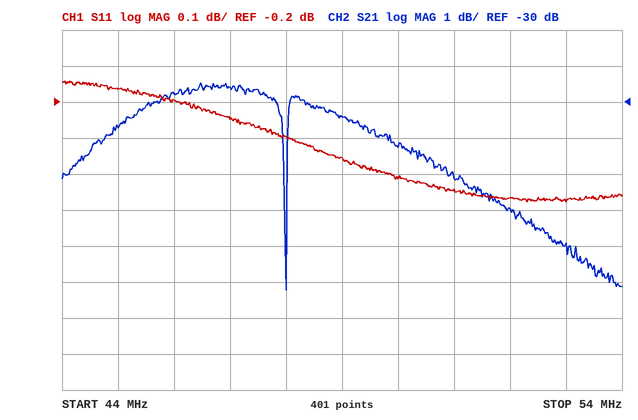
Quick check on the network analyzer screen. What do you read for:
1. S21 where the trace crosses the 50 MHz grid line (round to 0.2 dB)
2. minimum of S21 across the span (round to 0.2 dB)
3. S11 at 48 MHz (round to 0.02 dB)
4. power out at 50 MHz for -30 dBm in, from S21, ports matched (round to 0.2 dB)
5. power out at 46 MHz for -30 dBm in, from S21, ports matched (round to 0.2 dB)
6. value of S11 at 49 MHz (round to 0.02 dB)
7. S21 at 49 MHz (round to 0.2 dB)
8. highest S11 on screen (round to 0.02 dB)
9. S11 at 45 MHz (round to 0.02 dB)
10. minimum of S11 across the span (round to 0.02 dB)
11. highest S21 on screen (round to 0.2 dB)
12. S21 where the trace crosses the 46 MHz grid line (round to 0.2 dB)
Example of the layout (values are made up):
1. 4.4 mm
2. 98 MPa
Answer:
1. -31.2 dB
2. -35.2 dB
3. -0.30 dB
4. -61.2 dBm
5. -59.8 dBm
6. -0.36 dB
7. -30.4 dB
8. -0.14 dB
9. -0.16 dB
10. -0.48 dB
11. -29.4 dB
12. -29.8 dB
